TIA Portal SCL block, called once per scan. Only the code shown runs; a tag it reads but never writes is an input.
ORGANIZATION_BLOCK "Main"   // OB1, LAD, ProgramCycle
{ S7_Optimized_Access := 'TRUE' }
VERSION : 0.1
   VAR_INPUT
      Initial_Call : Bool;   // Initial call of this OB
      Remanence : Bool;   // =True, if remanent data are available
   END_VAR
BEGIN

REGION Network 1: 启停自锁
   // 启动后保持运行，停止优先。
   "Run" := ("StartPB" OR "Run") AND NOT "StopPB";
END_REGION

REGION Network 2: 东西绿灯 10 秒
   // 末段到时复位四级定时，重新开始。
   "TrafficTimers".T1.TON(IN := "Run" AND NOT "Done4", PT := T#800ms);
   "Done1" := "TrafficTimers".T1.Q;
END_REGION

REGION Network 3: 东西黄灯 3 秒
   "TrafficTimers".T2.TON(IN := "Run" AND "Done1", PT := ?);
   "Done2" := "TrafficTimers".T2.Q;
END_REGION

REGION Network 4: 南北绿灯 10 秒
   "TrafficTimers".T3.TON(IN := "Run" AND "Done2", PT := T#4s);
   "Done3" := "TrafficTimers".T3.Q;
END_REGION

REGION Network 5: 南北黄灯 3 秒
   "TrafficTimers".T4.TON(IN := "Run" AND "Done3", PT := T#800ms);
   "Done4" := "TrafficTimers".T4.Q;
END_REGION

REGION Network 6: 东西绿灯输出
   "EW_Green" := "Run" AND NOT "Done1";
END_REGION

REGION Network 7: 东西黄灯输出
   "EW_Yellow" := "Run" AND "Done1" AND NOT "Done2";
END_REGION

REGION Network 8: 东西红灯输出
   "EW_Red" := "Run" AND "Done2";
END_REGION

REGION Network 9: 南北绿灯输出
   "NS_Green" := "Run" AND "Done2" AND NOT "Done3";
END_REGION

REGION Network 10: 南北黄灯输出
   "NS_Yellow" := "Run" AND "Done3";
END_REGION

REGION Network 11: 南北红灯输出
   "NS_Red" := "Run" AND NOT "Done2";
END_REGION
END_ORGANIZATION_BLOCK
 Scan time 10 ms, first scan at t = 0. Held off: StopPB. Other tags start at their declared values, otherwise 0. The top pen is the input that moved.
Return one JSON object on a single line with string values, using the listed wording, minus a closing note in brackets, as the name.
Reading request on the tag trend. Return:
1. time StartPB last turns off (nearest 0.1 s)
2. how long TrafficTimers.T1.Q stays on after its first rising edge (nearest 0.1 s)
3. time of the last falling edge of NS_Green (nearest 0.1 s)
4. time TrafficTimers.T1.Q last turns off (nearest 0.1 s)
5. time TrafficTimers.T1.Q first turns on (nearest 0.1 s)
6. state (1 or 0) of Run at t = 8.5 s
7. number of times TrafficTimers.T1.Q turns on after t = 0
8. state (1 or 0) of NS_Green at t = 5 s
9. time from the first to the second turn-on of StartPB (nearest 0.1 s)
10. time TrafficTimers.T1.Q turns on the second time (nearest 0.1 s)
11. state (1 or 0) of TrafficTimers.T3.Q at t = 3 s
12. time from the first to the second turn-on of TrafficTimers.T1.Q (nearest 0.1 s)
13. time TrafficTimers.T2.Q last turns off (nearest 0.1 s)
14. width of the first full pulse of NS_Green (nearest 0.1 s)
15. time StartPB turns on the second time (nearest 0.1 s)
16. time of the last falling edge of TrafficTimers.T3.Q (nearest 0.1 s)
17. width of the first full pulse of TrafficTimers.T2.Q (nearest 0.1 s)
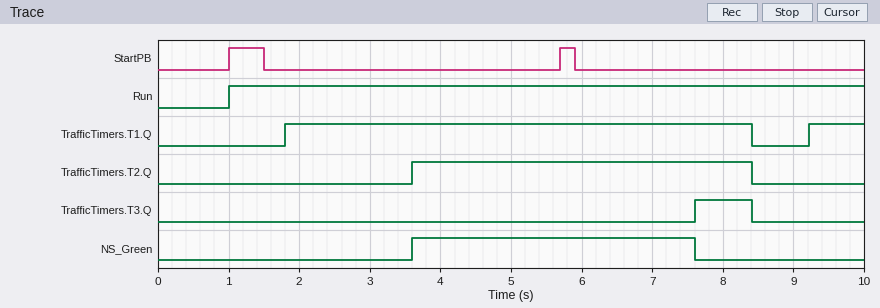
{"time StartPB last turns off": "5.9 s", "how long TrafficTimers.T1.Q stays on after its first rising edge": "6.6 s", "time of the last falling edge of NS_Green": "7.6 s", "time TrafficTimers.T1.Q last turns off": "8.4 s", "time TrafficTimers.T1.Q first turns on": "1.8 s", "state (1 or 0) of Run at t = 8.5 s": "1", "number of times TrafficTimers.T1.Q turns on after t = 0": "2", "state (1 or 0) of NS_Green at t = 5 s": "1", "time from the first to the second turn-on of StartPB": "4.7 s", "time TrafficTimers.T1.Q turns on the second time": "9.2 s", "state (1 or 0) of TrafficTimers.T3.Q at t = 3 s": "0", "time from the first to the second turn-on of TrafficTimers.T1.Q": "7.4 s", "time TrafficTimers.T2.Q last turns off": "8.4 s", "width of the first full pulse of NS_Green": "4.0 s", "time StartPB turns on the second time": "5.7 s", "time of the last falling edge of TrafficTimers.T3.Q": "8.4 s", "width of the first full pulse of TrafficTimers.T2.Q": "4.8 s"}
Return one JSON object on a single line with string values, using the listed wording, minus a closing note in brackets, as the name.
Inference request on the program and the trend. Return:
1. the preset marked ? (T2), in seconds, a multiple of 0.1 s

{"the preset marked ? (T2), in seconds, a multiple of 0.1 s": "1.8 s"}
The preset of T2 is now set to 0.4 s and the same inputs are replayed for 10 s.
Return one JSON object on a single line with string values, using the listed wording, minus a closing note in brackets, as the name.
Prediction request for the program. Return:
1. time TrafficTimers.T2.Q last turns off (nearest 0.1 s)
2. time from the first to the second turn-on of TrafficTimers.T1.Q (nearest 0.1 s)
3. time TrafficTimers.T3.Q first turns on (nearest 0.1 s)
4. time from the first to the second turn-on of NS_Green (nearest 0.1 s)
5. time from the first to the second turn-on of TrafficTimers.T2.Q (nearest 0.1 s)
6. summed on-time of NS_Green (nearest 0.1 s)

{"time TrafficTimers.T2.Q last turns off": "7.0 s", "time from the first to the second turn-on of TrafficTimers.T1.Q": "6.0 s", "time TrafficTimers.T3.Q first turns on": "6.2 s", "time from the first to the second turn-on of NS_Green": "6.0 s", "time from the first to the second turn-on of TrafficTimers.T2.Q": "6.0 s", "summed on-time of NS_Green": "5.8 s"}
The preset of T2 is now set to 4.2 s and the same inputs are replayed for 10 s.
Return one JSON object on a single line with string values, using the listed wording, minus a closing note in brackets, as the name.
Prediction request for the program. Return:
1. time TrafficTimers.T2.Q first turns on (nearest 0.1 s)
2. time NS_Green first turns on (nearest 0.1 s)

{"time TrafficTimers.T2.Q first turns on": "6.0 s", "time NS_Green first turns on": "6.0 s"}
